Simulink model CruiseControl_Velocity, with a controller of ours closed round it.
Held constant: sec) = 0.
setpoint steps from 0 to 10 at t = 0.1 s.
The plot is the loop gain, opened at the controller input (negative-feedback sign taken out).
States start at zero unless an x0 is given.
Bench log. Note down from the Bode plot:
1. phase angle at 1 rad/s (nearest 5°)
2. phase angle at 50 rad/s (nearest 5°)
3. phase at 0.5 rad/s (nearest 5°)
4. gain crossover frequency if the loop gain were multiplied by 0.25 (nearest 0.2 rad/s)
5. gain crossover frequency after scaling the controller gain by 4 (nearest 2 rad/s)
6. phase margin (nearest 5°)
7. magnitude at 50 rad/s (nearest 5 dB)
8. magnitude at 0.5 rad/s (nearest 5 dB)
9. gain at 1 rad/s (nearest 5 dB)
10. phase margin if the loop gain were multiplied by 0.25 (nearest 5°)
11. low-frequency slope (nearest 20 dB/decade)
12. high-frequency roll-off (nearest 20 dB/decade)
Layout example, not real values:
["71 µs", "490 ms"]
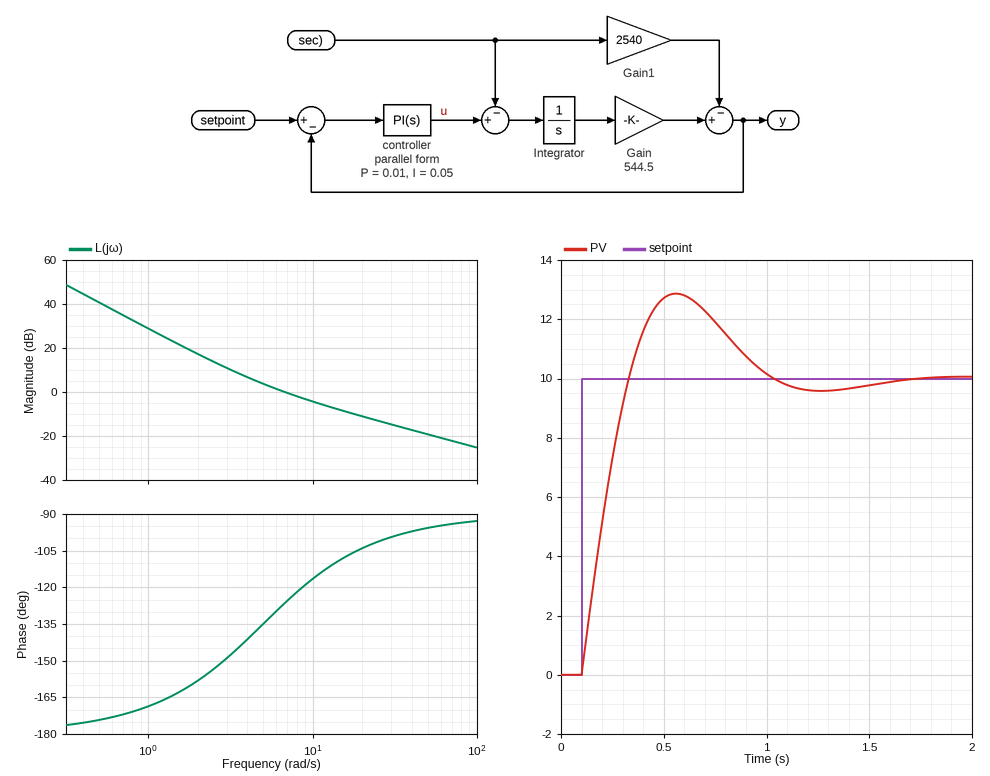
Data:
["-170°", "-95°", "-175°", "2.8 rad/s", "22 rad/s", "55°", "-20 dB", "40 dB", "30 dB", "30°", "-40 dB/decade", "-20 dB/decade"]
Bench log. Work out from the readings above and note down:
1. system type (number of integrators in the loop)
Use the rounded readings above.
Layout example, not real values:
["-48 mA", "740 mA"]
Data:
["2"]
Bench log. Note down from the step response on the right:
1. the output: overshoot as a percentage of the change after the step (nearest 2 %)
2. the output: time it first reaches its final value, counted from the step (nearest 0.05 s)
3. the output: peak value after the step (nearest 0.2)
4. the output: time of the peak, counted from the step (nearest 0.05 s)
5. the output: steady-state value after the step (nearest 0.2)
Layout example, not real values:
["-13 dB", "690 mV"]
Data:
["28 %", "0.25 s", "12.8", "0.45 s", "10.0"]
